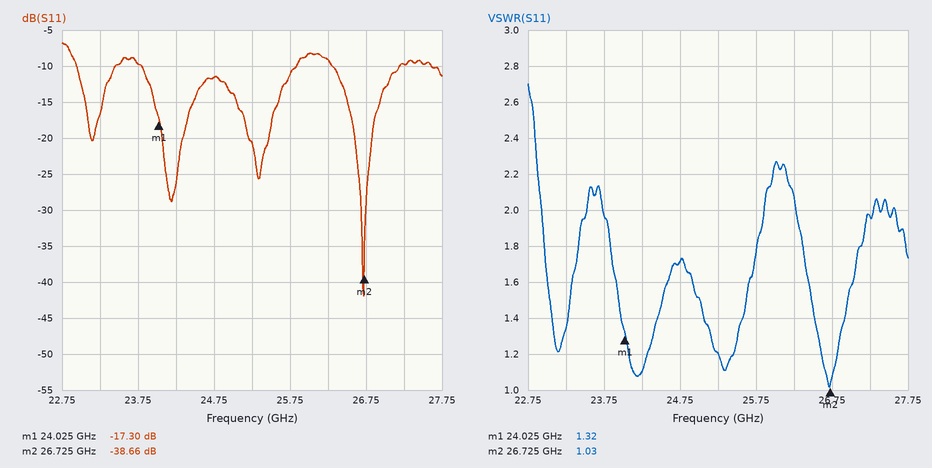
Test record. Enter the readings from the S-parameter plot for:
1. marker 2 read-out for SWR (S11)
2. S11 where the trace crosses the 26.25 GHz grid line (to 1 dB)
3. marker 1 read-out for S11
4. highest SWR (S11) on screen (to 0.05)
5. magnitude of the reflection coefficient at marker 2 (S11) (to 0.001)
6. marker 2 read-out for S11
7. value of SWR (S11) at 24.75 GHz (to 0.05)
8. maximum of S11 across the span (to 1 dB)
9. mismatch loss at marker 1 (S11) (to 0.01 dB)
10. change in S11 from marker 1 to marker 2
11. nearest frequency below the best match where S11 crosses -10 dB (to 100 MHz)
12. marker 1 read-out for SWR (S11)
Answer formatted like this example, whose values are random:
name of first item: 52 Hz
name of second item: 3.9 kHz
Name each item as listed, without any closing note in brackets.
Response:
marker 2 read-out for SWR: 1.03
S11 where the trace crosses the 26.25 GHz grid line: -9 dB
marker 1 read-out for S11: -17.30 dB
highest SWR (S11) on screen: 2.70
magnitude of the reflection coefficient at marker 2 (S11): 0.012
marker 2 read-out for S11: -38.66 dB
value of SWR (S11) at 24.75 GHz: 1.70
maximum of S11 across the span: -7 dB
mismatch loss at marker 1 (S11): 0.08 dB
change in S11 from marker 1 to marker 2: -21.36 dB
nearest frequency below the best match where S11 crosses -10 dB: 26.3 GHz
marker 1 read-out for SWR: 1.32
